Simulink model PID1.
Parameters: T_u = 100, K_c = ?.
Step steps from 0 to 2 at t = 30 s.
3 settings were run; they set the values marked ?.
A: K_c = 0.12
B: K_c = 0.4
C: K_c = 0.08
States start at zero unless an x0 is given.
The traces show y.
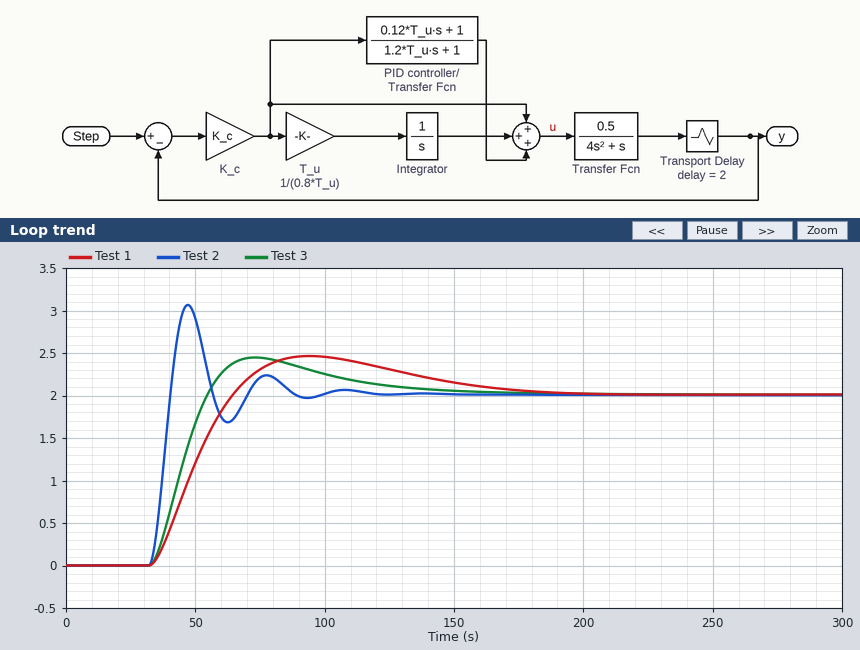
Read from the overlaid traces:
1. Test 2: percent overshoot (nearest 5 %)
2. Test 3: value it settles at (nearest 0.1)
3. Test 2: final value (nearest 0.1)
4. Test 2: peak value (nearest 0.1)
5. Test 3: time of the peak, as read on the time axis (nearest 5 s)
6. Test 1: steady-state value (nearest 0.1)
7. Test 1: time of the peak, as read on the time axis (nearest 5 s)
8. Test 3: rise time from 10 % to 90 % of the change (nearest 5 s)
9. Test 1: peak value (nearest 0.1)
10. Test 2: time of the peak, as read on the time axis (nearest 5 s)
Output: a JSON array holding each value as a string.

["55 %", "2.0", "2.0", "3.1", "75 s", "2.0", "95 s", "15 s", "2.5", "45 s"]
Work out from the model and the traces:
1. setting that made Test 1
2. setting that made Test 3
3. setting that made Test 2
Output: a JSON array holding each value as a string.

["C", "A", "B"]
